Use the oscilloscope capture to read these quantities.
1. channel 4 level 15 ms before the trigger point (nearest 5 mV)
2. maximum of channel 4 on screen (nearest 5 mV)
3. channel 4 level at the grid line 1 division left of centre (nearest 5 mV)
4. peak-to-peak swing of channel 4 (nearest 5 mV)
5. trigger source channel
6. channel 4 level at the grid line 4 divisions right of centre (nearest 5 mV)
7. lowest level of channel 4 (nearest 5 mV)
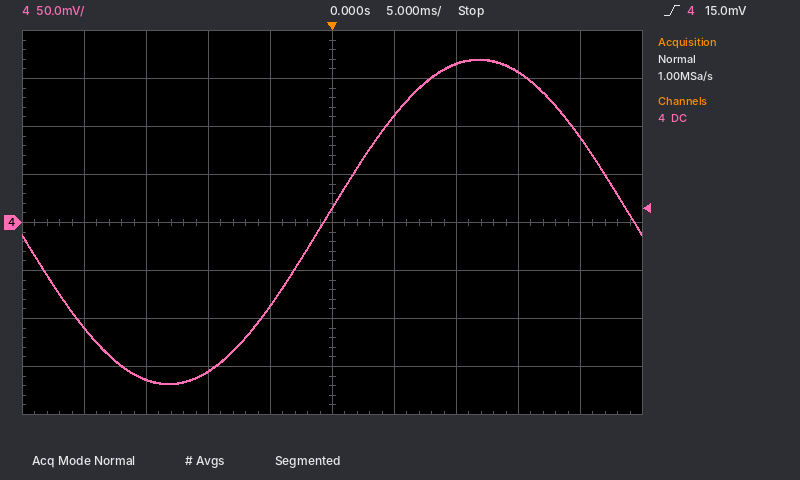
-165 mV
170 mV
-85 mV
340 mV
channel 4
90 mV
-170 mV
